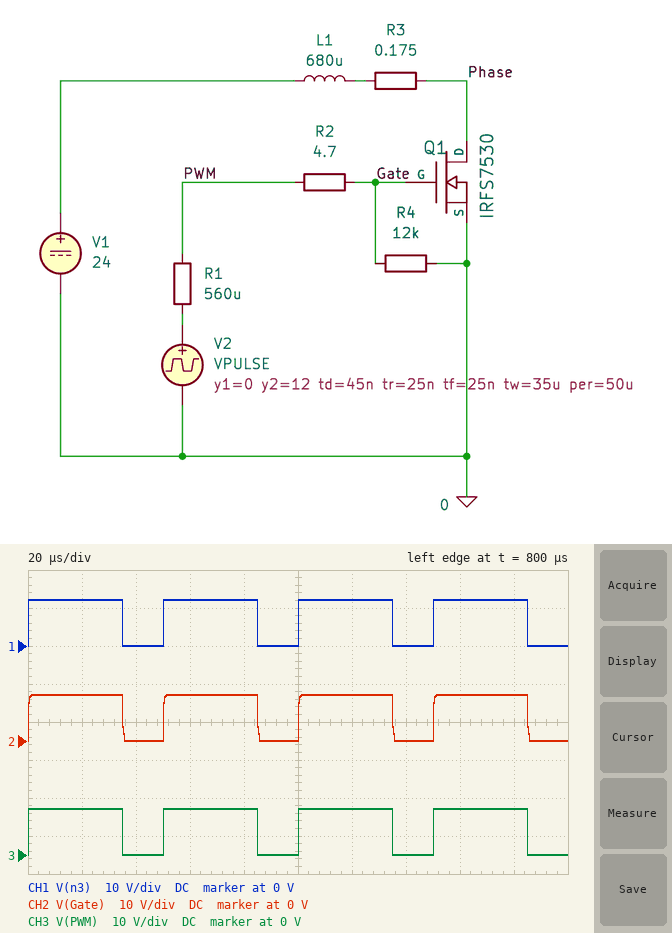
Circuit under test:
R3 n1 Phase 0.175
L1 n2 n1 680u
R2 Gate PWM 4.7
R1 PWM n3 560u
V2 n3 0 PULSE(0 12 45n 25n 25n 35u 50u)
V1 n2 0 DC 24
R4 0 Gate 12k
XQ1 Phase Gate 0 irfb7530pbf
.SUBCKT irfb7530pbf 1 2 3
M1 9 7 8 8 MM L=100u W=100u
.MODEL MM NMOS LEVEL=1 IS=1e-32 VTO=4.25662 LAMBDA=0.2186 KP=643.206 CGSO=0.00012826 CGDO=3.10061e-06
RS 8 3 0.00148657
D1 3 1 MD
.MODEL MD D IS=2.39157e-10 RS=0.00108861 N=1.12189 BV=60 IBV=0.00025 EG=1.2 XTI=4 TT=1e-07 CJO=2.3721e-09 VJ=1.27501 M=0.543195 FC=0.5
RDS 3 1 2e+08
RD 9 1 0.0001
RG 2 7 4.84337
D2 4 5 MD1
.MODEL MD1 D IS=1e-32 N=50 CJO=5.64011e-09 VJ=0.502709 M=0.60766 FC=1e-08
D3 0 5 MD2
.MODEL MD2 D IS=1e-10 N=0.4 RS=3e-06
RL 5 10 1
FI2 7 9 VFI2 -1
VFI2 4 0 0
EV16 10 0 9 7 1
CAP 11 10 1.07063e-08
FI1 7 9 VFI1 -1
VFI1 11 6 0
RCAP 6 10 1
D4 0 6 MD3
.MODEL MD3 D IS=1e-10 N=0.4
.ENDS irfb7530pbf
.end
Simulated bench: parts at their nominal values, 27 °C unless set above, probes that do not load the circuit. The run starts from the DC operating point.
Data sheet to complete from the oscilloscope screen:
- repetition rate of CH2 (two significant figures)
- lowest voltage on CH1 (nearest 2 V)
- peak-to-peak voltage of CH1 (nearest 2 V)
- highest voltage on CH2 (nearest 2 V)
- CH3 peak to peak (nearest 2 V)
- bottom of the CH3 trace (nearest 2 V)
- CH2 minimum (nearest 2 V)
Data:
20 kHz
0 V
12 V
12 V
12 V
0 V
0 V
